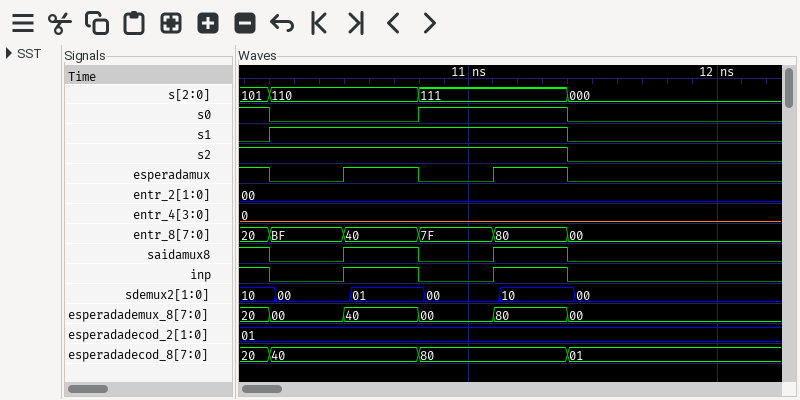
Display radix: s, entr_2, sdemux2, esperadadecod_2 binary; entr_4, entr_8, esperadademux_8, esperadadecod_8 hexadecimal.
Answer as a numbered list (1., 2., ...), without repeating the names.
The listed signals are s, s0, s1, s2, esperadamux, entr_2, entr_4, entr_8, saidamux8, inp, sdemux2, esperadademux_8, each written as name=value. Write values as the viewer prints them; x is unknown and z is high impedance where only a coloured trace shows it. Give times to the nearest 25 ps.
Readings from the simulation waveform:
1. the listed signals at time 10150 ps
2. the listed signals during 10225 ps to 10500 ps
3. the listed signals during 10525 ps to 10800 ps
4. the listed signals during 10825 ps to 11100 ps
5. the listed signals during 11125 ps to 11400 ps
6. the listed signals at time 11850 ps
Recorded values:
1. s=101, s0=1, s1=0, s2=1, esperadamux=1, entr_2=00, entr_4=0, entr_8=20, saidamux8=1, inp=1, sdemux2=10, esperadademux_8=20
2. s=110, s0=0, s1=1, s2=1, esperadamux=0, entr_2=00, entr_4=0, entr_8=BF, saidamux8=0, inp=0, sdemux2=00, esperadademux_8=00
3. s=110, s0=0, s1=1, s2=1, esperadamux=1, entr_2=00, entr_4=0, entr_8=40, saidamux8=1, inp=1, sdemux2=01, esperadademux_8=40
4. s=111, s0=1, s1=1, s2=1, esperadamux=0, entr_2=00, entr_4=0, entr_8=7F, saidamux8=0, inp=0, sdemux2=00, esperadademux_8=00
5. s=111, s0=1, s1=1, s2=1, esperadamux=1, entr_2=00, entr_4=0, entr_8=80, saidamux8=1, inp=1, sdemux2=10, esperadademux_8=80
6. s=000, s0=0, s1=0, s2=0, esperadamux=0, entr_2=00, entr_4=0, entr_8=00, saidamux8=0, inp=0, sdemux2=00, esperadademux_8=00
